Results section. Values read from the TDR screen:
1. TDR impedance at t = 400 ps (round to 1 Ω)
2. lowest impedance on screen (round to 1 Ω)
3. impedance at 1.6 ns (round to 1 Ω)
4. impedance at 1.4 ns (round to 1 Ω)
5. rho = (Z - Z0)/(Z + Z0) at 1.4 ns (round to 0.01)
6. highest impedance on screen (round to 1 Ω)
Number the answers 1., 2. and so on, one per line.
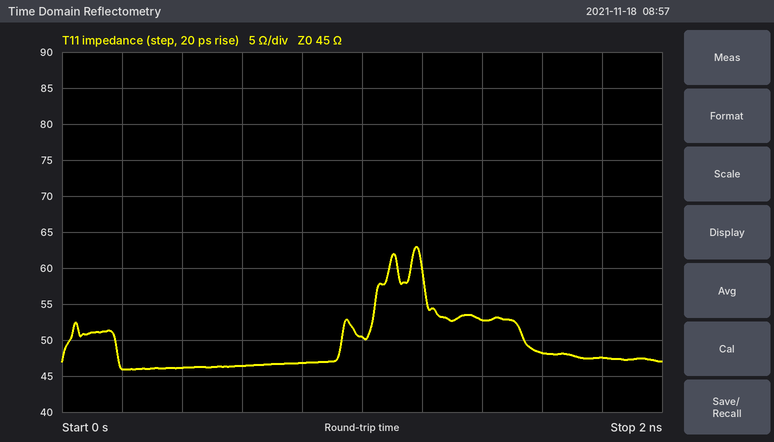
1. 46 Ω
2. 46 Ω
3. 48 Ω
4. 53 Ω
5. +0.08
6. 63 Ω
